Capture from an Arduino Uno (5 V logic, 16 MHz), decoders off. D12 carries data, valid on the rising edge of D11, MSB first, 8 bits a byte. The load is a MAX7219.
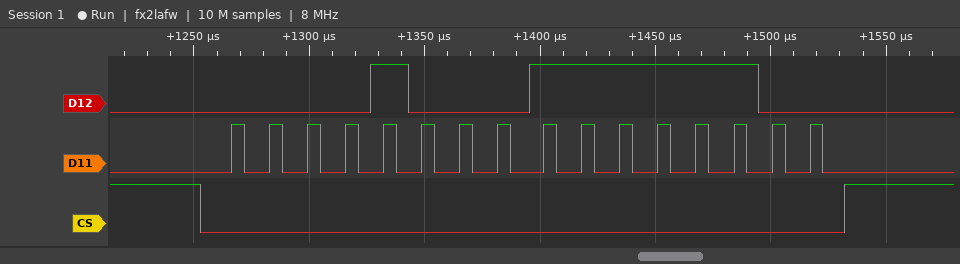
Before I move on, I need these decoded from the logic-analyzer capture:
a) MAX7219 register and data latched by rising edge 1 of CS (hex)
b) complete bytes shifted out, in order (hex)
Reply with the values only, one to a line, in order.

register 0x8, data 0xFC
08 FC
